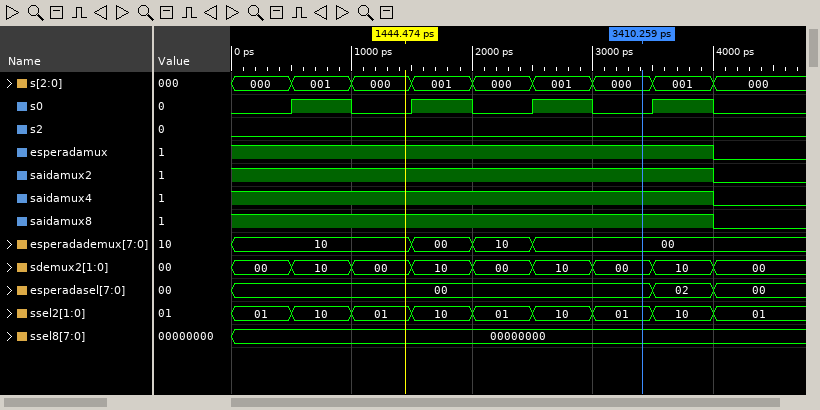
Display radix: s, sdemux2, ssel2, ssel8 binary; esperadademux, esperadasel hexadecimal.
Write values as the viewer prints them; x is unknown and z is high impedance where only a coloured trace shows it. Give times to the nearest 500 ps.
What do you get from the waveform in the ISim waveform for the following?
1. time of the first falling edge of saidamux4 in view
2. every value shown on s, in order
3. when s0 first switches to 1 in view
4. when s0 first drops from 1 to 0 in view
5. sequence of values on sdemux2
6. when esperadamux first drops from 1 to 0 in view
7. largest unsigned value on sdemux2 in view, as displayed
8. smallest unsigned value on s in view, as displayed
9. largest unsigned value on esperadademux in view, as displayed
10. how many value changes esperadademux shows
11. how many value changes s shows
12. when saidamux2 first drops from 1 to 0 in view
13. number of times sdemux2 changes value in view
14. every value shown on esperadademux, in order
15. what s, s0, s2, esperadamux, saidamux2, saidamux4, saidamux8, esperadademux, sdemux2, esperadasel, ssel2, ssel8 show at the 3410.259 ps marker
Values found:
4000 ps
000, 001, 000, 001, 000, 001, 000, 001, 000
500 ps
1000 ps
00, 10, 00, 10, 00, 10, 00, 10, 00
4000 ps
10
000
10
3
8
4000 ps
8
10, 00, 10, 00
s=000, s0=0, s2=0, esperadamux=1, saidamux2=1, saidamux4=1, saidamux8=1, esperadademux=00, sdemux2=00, esperadasel=00, ssel2=01, ssel8=00000000
